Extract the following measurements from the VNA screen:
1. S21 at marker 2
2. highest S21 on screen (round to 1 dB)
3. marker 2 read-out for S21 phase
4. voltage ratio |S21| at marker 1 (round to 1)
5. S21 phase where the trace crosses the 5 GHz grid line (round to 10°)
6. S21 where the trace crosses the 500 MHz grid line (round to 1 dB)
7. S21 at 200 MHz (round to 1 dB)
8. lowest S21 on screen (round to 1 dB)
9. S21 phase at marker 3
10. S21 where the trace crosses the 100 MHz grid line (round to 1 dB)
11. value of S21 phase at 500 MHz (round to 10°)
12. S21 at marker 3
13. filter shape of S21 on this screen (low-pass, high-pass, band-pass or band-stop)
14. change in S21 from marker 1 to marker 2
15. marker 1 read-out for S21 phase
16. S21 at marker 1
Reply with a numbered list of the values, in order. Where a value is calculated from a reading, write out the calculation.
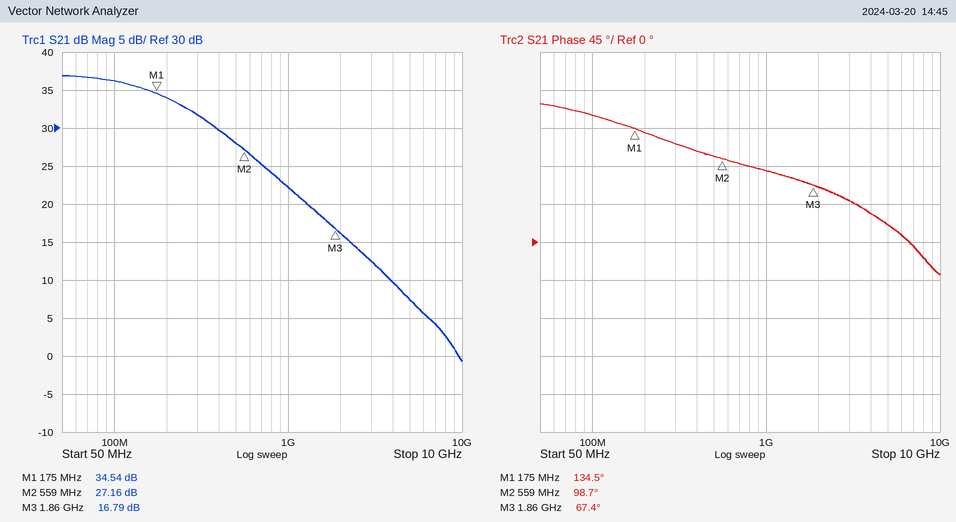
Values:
1. 27.16 dB
2. 37 dB
3. 98.7°
4. 10^(34.54/20) ≈ 53
5. 20°
6. 28 dB
7. 34 dB
8. -1 dB
9. 67.4°
10. 36 dB
11. 100°
12. 16.79 dB
13. low-pass
14. 27.16 − (34.54) = -7.38 dB
15. 134.5°
16. 34.54 dB
